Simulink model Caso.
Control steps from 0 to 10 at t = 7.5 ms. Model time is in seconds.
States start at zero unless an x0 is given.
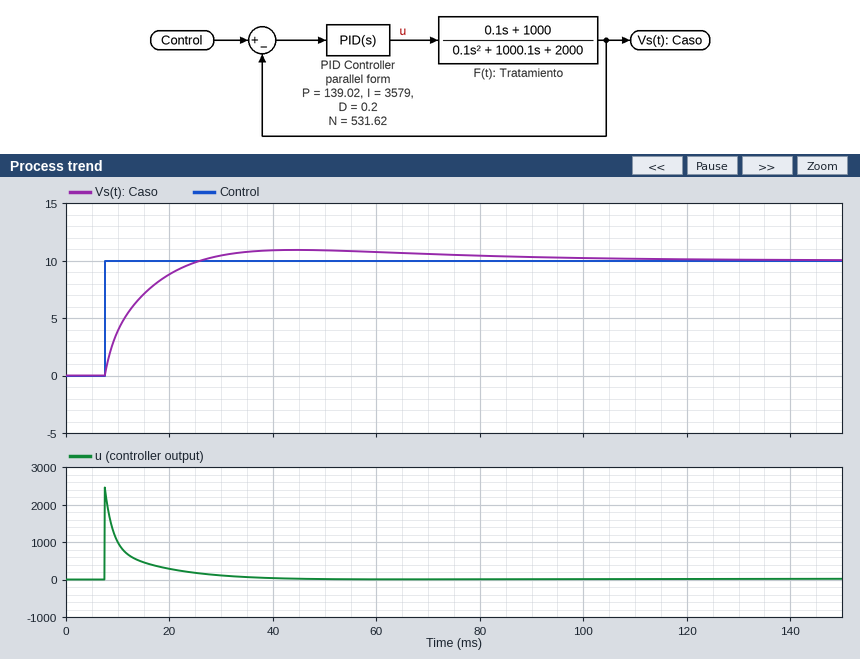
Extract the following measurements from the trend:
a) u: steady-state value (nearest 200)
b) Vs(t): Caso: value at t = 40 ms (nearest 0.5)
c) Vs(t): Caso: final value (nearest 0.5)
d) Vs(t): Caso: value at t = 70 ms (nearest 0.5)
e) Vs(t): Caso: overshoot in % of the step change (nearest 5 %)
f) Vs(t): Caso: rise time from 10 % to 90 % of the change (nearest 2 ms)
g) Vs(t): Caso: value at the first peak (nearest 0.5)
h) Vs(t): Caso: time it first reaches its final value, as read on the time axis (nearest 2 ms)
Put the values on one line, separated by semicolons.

0; 11.0; 10.0; 10.5; 10 %; 12 ms; 11.0; 26 ms
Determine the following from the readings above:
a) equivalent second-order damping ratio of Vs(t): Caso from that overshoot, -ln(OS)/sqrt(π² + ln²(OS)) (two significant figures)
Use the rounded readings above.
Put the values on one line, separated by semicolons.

0.59
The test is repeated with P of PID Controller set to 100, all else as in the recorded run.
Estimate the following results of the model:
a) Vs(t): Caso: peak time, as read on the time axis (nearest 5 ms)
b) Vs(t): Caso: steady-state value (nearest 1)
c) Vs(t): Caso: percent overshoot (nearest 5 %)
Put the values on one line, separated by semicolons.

50 ms; 10; 15 %
